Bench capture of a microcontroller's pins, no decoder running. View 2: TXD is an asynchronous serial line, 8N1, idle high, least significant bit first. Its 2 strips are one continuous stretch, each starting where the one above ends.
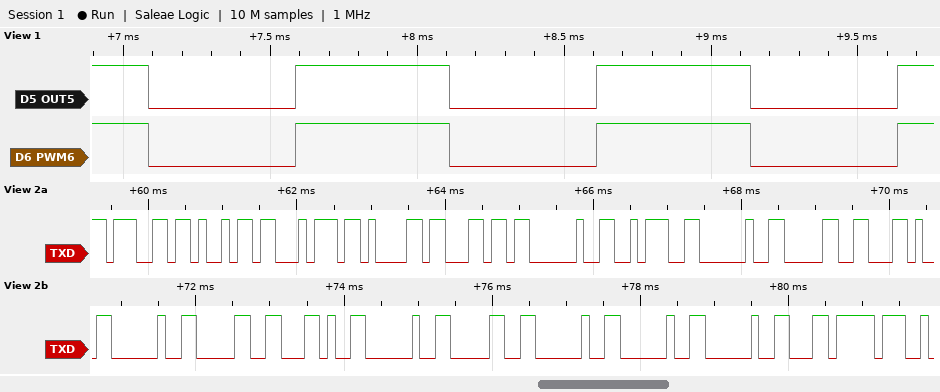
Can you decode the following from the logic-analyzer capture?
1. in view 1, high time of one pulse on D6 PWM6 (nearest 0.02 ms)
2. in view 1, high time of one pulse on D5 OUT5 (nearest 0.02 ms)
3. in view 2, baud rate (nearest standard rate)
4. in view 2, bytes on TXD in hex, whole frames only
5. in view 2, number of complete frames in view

0.52 ms
0.52 ms
9600 baud
67 69 74 61 6C 20 3A 20 30 2C 20 30 2C 20 30 20 20 20 EC
19
